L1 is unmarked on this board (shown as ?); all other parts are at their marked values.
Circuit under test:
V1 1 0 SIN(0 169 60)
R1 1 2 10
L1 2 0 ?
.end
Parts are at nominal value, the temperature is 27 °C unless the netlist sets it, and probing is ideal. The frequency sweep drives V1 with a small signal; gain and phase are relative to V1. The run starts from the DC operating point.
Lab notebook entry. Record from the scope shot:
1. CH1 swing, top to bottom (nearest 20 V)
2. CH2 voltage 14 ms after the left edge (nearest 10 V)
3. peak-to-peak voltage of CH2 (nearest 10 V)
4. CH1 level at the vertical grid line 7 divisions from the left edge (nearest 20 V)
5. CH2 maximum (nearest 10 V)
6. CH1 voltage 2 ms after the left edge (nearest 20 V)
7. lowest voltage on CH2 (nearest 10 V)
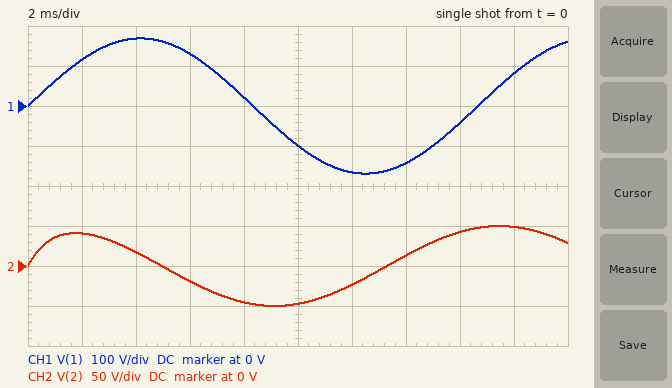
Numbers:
340 V
10 V
100 V
-140 V
50 V
120 V
-50 V
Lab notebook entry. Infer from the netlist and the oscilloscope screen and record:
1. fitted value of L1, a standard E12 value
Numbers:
8.2 mH
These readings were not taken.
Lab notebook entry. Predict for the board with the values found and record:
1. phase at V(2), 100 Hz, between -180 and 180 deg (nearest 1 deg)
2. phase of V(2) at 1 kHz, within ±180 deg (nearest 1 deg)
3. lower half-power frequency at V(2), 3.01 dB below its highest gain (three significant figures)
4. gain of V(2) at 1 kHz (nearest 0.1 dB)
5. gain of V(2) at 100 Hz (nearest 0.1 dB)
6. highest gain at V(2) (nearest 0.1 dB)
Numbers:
63 deg
11 deg
194 Hz
-0.2 dB
-6.8 dB
0 dB
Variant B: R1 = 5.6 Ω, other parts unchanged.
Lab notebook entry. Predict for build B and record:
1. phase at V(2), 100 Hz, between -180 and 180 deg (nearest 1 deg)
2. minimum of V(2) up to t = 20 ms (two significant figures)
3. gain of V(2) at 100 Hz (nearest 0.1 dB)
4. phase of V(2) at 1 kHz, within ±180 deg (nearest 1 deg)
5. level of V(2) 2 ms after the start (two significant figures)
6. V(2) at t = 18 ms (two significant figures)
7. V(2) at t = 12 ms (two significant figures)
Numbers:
47 deg
-82 V
-3.4 dB
6 deg
61 V
82 V
-52 V
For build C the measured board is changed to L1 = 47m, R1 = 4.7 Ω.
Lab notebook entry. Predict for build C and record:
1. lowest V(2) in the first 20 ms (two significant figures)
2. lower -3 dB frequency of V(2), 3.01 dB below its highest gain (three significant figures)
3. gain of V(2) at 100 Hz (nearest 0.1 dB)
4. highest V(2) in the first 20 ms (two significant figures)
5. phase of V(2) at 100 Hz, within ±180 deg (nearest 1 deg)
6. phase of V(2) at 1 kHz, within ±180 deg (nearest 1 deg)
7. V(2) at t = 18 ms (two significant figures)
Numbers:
-180 V
15.9 Hz
-0.1 dB
160 V
9 deg
1 deg
110 V
